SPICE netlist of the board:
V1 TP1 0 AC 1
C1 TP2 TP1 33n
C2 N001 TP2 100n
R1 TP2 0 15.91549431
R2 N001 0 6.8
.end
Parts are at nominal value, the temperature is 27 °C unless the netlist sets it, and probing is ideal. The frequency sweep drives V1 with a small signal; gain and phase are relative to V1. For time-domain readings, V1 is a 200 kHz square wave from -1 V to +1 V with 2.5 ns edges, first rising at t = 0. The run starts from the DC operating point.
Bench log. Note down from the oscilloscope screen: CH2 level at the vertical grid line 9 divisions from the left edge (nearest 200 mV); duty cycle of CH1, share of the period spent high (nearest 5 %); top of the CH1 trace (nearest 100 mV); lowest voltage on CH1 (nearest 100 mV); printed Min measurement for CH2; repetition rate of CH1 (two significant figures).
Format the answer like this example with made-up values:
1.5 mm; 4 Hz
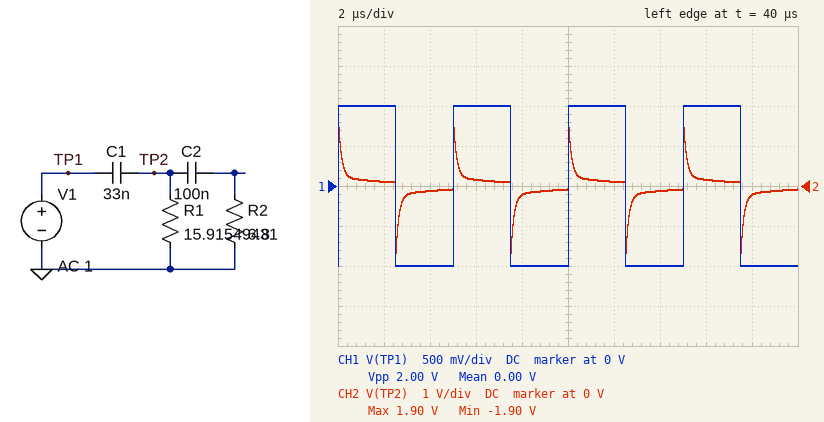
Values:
-200 mV; 50 %; 1.0 V; -1.0 V; -1.90 V; 200 kHz
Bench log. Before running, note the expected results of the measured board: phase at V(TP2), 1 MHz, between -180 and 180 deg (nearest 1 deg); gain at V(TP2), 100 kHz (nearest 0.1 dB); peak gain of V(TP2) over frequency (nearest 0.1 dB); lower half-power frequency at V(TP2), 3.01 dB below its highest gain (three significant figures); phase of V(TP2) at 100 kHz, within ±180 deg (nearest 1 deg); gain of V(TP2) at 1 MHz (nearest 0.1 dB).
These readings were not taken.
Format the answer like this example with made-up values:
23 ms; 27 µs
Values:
40 deg; -14.7 dB; 0 dB; 1.14 MHz; 49 deg; -3.6 dB
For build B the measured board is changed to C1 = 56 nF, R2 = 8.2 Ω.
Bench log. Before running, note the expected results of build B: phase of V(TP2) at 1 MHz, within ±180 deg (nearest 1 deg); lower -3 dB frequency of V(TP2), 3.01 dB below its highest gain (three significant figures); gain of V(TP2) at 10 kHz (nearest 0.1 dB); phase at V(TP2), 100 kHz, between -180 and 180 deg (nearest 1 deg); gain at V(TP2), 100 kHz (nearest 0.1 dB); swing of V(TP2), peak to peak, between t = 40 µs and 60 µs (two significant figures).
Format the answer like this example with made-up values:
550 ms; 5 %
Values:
26 deg; 613 kHz; -25.2 dB; 46 deg; -10.8 dB; 3.7 V
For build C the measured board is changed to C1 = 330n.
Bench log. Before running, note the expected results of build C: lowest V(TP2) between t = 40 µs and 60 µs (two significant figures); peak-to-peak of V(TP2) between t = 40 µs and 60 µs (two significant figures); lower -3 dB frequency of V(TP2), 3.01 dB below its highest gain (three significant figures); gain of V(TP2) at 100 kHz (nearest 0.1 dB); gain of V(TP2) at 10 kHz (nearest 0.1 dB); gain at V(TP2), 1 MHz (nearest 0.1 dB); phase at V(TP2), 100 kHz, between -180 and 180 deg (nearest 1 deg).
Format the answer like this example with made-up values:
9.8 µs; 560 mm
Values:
-1.4 V; 2.8 V; 58.4 kHz; -2.4 dB; -10.4 dB; -0.2 dB; 18 deg
